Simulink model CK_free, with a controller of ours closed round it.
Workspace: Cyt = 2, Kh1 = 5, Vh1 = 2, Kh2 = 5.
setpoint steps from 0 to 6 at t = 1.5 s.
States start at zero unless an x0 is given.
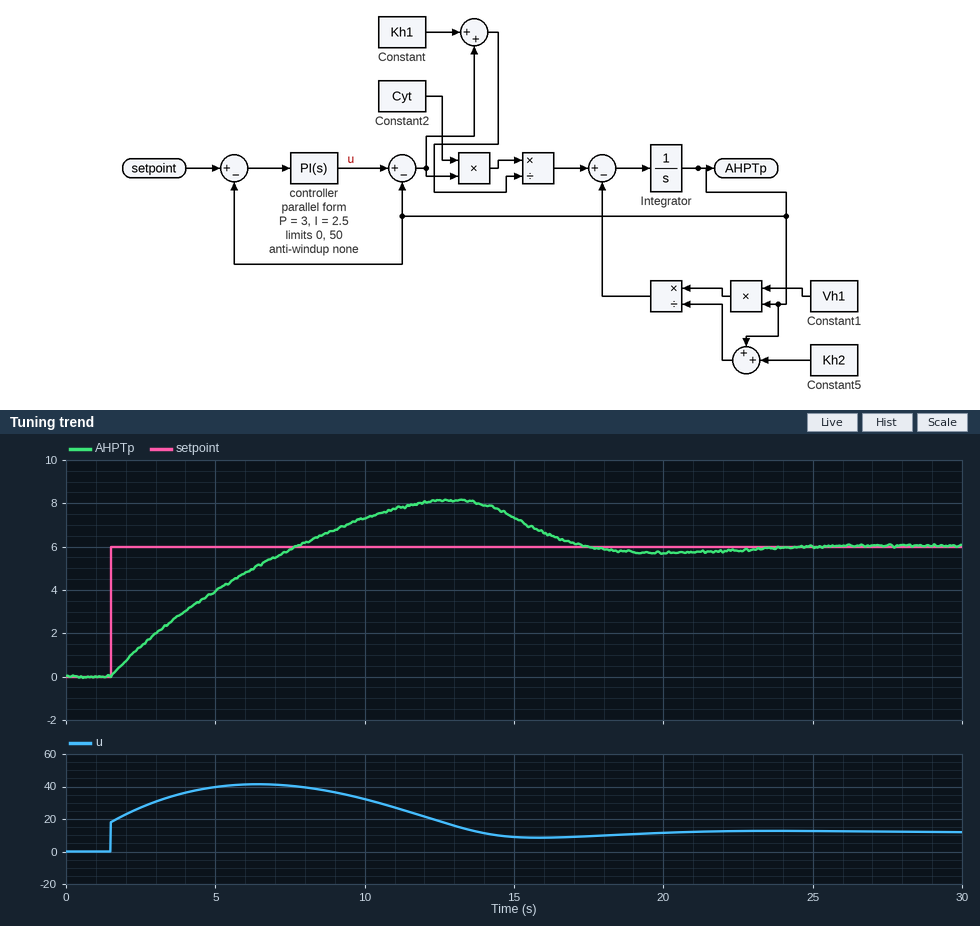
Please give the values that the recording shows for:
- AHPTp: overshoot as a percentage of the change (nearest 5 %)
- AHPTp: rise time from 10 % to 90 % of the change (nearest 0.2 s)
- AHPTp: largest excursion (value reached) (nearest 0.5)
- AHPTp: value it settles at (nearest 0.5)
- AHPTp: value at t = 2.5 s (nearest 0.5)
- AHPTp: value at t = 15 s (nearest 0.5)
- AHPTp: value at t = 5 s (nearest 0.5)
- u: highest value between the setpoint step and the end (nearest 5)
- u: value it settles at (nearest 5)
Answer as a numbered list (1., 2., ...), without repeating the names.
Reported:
1. 35 %
2. 5.0 s
3. 8.0
4. 6.0
5. 1.5
6. 7.5
7. 4.0
8. 40
9. 10
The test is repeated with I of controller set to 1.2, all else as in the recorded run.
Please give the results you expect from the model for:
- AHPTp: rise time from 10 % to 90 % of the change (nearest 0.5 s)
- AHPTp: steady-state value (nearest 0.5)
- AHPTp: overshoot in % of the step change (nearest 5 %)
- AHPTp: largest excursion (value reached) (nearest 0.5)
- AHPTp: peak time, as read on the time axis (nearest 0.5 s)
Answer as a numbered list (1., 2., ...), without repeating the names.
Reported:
1. 6.0 s
2. 6.0
3. 20 %
4. 7.0
5. 14.0 s
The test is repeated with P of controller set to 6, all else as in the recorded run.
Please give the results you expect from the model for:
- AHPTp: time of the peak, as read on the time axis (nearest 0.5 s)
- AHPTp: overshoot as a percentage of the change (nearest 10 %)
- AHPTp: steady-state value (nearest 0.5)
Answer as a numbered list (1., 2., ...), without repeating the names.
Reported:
1. 12.0 s
2. 30 %
3. 6.0
